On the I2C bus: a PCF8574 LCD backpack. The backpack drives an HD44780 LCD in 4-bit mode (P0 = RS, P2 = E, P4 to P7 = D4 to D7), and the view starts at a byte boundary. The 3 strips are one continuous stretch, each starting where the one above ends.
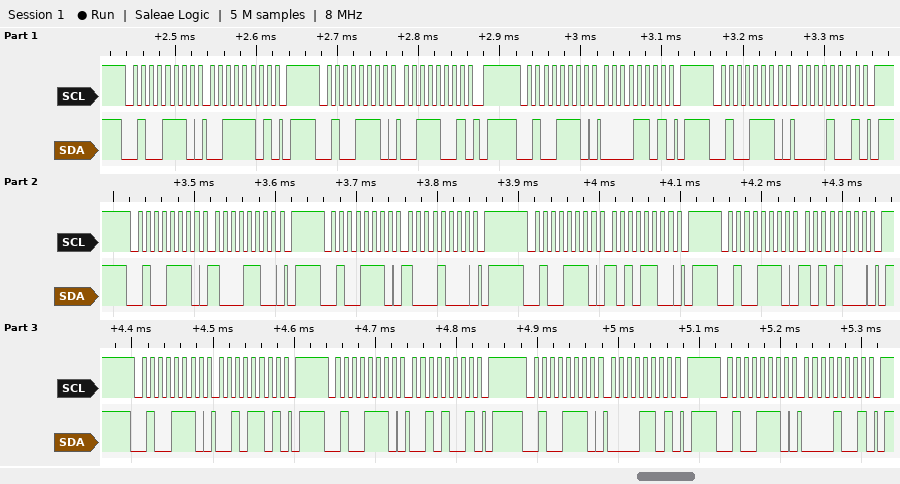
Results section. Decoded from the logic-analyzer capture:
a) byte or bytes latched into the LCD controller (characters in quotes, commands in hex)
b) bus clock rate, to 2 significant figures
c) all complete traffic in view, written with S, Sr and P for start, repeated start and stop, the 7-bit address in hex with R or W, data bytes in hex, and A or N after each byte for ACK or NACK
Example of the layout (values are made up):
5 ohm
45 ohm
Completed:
'0' 0x8A ' '
100 kHz
S 27W A 3D A P S 27W A 39 A P S 27W A 0D A P S 27W A 09 A P S 27W A 8C A P S 27W A 88 A P S 27W A AC A P S 27W A A8 A P S 27W A 2D A P S 27W A 29 A P S 27W A 0D A P S 27W A 09 A P
